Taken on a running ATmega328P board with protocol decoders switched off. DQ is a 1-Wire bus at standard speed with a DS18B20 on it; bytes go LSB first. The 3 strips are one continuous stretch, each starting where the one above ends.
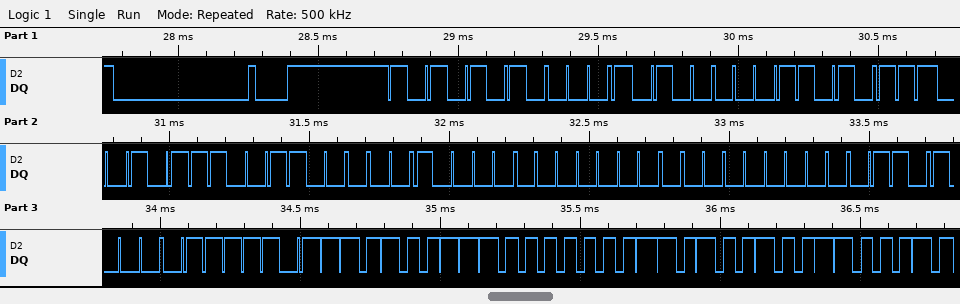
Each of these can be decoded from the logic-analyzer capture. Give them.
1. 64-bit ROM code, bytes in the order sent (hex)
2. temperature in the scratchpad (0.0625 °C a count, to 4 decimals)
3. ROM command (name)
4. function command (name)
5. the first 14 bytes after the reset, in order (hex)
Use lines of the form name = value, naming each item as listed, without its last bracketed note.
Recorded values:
64-bit ROM code, bytes in the order sent = 28 58 A7 33 08 00 00 16
temperature in the scratchpad = 28.6875 °C
ROM command = Match ROM
function command = Read Scratchpad
the first 14 bytes after the reset, in order = 55 28 58 A7 33 08 00 00 16 BE CB 01 4B 46
